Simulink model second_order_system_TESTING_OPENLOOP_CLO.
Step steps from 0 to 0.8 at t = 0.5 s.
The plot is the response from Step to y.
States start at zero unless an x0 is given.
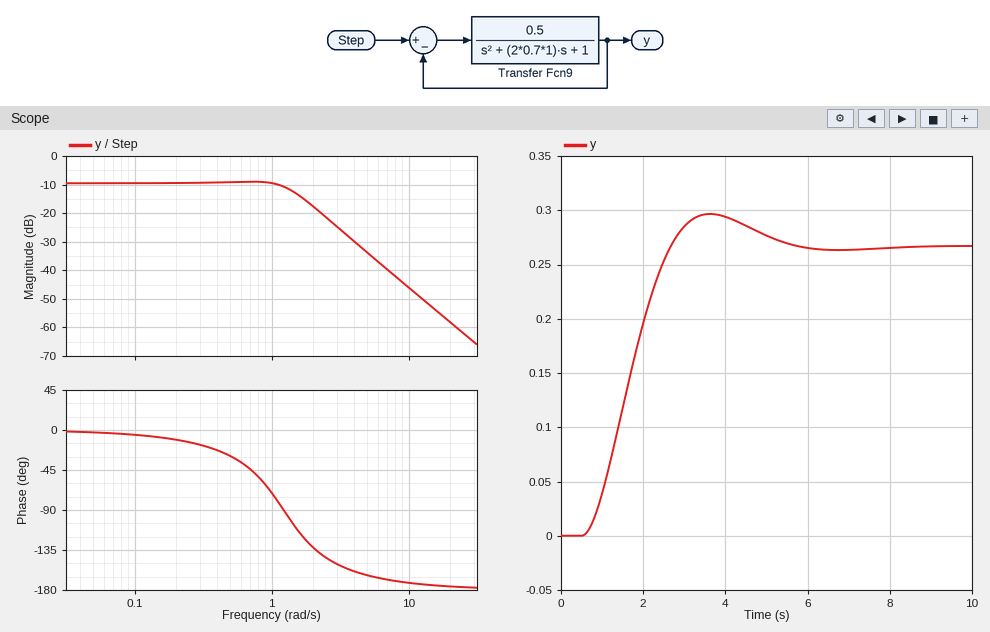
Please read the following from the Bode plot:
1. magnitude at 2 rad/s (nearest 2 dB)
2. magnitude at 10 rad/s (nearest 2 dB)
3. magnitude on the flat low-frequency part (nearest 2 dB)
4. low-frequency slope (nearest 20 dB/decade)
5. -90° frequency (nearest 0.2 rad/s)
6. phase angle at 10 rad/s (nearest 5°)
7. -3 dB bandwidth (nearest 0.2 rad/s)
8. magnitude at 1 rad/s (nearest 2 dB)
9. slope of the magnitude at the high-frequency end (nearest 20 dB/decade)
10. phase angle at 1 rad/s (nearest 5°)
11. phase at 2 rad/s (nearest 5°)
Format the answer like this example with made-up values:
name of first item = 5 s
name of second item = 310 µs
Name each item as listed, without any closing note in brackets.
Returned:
magnitude at 2 rad/s = -18 dB
magnitude at 10 rad/s = -46 dB
magnitude on the flat low-frequency part = -10 dB
low-frequency slope = 0 dB/decade
-90° frequency = 1.2 rad/s
phase angle at 10 rad/s = -170°
-3 dB bandwidth = 1.4 rad/s
magnitude at 1 rad/s = -10 dB
slope of the magnitude at the high-frequency end = -40 dB/decade
phase angle at 1 rad/s = -70°
phase at 2 rad/s = -130°
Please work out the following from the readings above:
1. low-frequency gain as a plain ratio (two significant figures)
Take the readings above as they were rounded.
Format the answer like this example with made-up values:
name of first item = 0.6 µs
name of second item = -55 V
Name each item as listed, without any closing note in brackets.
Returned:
low-frequency gain as a plain ratio = 0.32
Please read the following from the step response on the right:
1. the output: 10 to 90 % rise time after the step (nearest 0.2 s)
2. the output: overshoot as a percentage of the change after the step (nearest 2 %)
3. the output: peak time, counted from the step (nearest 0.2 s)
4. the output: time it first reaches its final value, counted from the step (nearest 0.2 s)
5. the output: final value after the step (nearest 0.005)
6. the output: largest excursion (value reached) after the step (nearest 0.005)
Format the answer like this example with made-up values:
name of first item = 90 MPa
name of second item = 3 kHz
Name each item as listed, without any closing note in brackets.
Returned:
the output: 10 to 90 % rise time after the step = 1.4 s
the output: overshoot as a percentage of the change after the step = 12 %
the output: peak time, counted from the step = 3.2 s
the output: time it first reaches its final value, counted from the step = 2.2 s
the output: final value after the step = 0.265
the output: largest excursion (value reached) after the step = 0.295
